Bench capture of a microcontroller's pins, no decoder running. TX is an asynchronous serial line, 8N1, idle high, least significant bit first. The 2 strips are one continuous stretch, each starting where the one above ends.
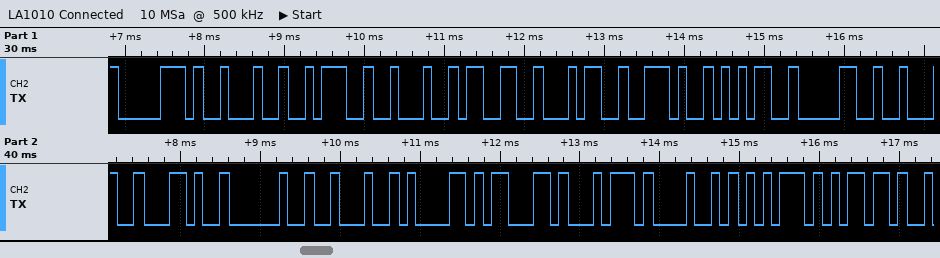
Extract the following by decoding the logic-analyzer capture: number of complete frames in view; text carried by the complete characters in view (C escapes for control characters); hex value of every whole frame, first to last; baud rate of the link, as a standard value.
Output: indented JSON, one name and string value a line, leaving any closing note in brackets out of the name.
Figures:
{
  "number of complete frames in view": "19",
  "text carried by the complete characters in view": "\"p\\\":\\\"34.50\\\", \\\"actHum\"",
  "hex value of every whole frame, first to last": "0x70 0x22 0x3A 0x22 0x33 0x34 0x2E 0x35 0x30 0x22 0x2C 0x20 0x22 0x61 0x63 0x74 0x48 0x75 0x6D",
  "baud rate of the link, as a standard value": "9600 baud"
}
